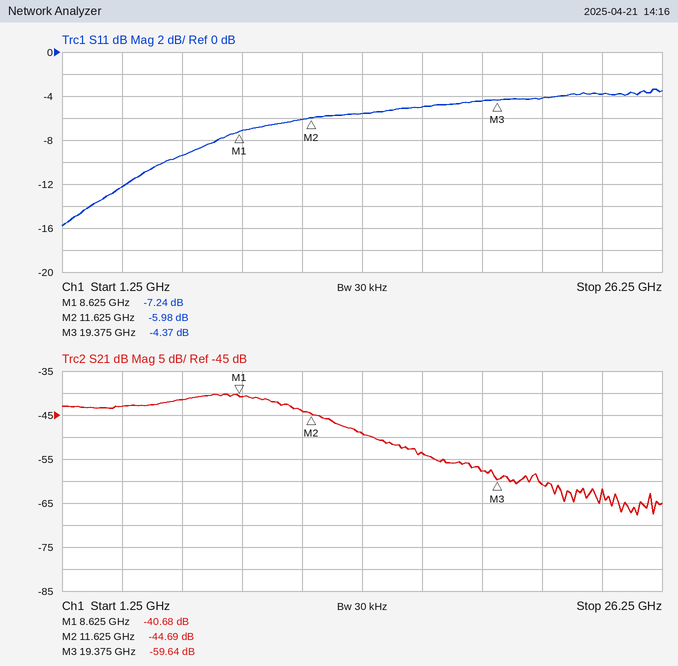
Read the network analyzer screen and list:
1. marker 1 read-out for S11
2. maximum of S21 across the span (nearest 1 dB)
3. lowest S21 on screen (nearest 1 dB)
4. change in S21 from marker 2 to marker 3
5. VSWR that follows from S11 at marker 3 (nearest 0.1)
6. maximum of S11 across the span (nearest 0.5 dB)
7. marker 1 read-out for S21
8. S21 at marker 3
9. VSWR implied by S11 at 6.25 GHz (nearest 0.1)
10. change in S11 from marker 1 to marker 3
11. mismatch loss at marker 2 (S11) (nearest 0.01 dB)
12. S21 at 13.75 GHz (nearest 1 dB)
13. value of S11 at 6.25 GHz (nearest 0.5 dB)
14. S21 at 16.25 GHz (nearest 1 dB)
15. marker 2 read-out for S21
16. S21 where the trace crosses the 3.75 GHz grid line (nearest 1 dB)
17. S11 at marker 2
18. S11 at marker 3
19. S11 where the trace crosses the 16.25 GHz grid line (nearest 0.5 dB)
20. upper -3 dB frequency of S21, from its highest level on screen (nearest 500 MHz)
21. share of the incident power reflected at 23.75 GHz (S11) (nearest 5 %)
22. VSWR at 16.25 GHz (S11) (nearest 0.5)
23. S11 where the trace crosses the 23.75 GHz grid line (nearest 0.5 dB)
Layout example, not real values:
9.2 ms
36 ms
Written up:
-7.24 dB
-40 dB
-68 dB
-14.95 dB
4.1
-3.5 dB
-40.68 dB
-59.64 dB
2.0
2.87 dB
1.26 dB
-49 dB
-9.5 dB
-54 dB
-44.69 dB
-43 dB
-5.98 dB
-4.37 dB
-5.0 dB
11.0 GHz
40 %
3.5
-4.0 dB
